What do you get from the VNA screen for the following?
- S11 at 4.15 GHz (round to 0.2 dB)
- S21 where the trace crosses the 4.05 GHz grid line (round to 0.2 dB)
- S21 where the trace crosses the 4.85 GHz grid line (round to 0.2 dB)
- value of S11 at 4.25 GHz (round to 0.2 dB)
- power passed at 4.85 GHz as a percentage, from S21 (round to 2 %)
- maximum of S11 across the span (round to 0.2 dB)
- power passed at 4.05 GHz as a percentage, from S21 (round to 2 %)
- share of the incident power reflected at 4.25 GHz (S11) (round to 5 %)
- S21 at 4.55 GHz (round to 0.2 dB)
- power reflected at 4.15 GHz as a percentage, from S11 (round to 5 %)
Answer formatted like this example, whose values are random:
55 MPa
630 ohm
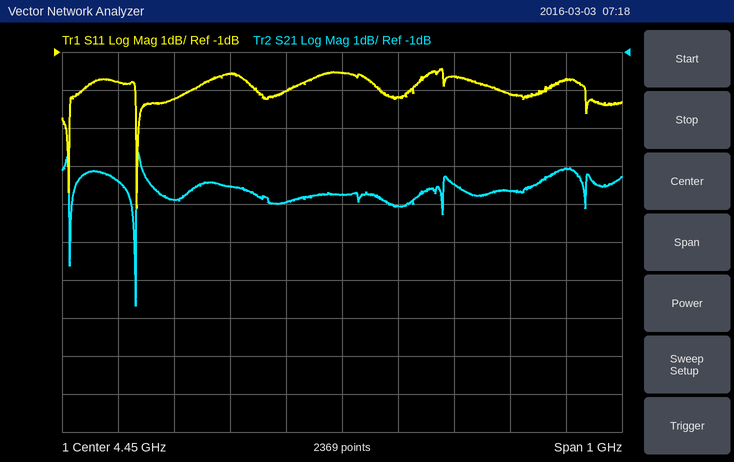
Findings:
-2.2 dB
-4.4 dB
-4.0 dB
-1.6 dB
40 %
-1.4 dB
36 %
70 %
-5.0 dB
60 %
